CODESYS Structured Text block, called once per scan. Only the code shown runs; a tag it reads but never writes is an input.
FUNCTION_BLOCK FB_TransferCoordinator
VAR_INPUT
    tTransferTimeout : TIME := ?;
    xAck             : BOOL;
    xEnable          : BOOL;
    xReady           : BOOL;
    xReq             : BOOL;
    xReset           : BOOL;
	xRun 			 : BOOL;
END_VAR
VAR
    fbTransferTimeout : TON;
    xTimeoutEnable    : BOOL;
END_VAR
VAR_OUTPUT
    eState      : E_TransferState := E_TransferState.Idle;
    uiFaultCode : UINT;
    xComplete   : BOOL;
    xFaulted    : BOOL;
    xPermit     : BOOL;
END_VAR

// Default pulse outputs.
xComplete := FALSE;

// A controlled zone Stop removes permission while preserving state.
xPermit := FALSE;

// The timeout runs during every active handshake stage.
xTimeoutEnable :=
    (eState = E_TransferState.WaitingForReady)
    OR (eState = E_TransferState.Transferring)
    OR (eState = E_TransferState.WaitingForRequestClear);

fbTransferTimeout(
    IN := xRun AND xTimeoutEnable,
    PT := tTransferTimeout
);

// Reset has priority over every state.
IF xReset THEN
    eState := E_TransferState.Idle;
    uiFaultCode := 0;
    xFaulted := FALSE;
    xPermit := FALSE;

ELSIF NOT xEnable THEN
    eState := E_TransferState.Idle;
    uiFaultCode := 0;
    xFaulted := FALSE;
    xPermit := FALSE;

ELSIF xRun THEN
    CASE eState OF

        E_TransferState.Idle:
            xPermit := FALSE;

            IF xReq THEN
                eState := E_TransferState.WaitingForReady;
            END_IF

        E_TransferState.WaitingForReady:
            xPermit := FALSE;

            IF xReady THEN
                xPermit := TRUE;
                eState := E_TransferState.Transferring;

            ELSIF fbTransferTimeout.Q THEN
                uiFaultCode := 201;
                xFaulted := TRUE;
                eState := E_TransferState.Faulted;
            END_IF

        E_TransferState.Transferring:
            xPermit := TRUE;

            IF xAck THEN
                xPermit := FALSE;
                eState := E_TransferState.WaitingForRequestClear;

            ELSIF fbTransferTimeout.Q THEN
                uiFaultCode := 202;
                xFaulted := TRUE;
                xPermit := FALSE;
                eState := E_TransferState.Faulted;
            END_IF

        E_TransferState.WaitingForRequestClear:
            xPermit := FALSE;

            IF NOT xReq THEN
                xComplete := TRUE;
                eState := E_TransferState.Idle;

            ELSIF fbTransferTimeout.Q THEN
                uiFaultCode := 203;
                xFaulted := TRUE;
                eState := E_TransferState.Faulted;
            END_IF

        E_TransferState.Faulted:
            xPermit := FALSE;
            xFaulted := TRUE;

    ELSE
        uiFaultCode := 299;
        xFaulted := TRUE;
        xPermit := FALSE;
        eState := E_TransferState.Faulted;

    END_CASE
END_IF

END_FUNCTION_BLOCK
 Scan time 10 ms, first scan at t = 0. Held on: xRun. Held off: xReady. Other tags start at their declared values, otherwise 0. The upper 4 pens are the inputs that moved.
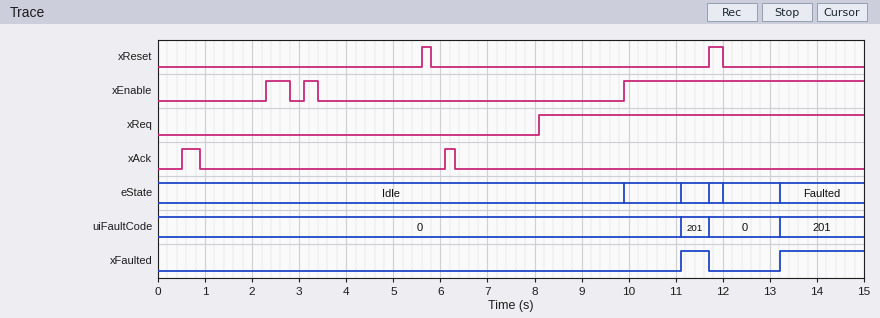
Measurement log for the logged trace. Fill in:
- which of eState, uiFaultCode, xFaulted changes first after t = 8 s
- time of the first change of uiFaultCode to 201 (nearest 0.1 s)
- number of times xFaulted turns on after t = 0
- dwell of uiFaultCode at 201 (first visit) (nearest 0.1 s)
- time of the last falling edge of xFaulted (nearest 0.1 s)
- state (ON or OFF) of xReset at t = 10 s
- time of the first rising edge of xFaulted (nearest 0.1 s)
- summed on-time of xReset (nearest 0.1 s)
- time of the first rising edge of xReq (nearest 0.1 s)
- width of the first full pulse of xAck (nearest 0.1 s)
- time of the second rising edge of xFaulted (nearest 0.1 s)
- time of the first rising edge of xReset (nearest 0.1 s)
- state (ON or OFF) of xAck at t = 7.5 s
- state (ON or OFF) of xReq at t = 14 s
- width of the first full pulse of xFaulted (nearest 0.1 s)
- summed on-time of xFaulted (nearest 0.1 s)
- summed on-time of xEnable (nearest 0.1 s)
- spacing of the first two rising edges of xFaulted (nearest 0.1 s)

eState
11.1 s
2
0.6 s
11.7 s
OFF
11.1 s
0.5 s
8.1 s
0.4 s
13.2 s
5.6 s
OFF
ON
0.6 s
2.4 s
5.9 s
2.1 s
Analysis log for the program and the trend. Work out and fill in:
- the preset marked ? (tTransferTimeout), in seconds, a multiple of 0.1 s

1.2 s
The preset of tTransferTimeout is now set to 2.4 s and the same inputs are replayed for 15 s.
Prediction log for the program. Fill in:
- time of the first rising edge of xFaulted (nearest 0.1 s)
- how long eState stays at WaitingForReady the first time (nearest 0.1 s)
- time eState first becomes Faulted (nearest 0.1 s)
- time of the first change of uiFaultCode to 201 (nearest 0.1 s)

14.4 s
1.8 s
14.4 s
14.4 s
